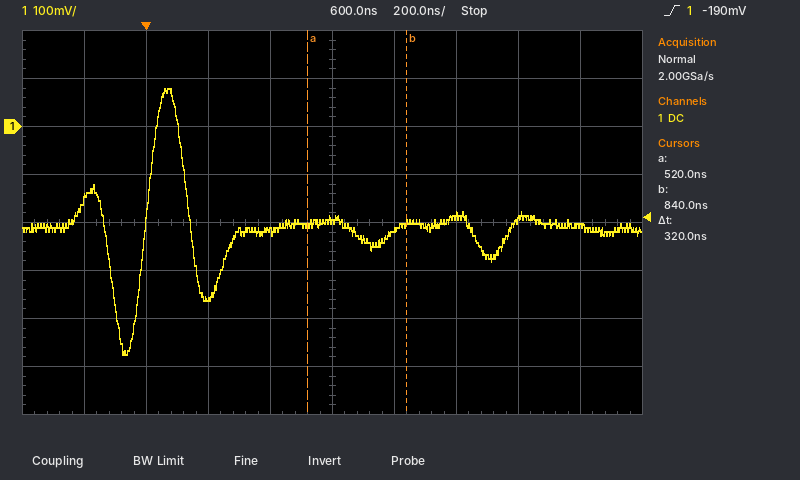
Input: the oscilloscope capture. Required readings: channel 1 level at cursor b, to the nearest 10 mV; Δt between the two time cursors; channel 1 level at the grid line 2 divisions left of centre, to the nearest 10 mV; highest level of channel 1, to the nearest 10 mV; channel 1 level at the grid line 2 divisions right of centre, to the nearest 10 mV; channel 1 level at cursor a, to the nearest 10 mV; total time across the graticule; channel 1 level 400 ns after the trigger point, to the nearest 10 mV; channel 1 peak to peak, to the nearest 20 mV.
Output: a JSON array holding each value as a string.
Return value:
["-200 mV", "320 ns", "-360 mV", "80 mV", "-190 mV", "-200 mV", "2 µs", "-220 mV", "560 mV"]
